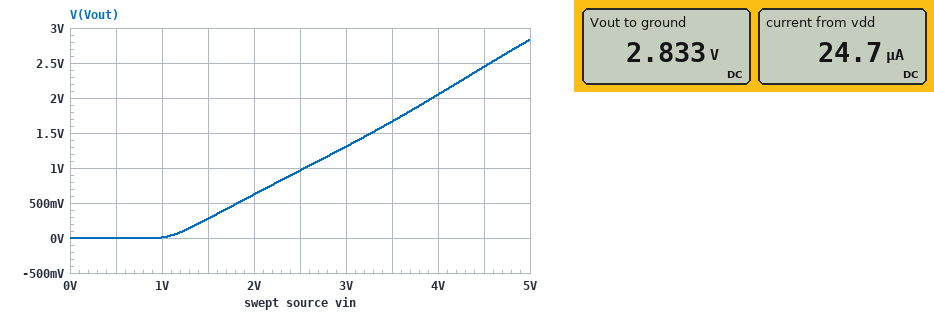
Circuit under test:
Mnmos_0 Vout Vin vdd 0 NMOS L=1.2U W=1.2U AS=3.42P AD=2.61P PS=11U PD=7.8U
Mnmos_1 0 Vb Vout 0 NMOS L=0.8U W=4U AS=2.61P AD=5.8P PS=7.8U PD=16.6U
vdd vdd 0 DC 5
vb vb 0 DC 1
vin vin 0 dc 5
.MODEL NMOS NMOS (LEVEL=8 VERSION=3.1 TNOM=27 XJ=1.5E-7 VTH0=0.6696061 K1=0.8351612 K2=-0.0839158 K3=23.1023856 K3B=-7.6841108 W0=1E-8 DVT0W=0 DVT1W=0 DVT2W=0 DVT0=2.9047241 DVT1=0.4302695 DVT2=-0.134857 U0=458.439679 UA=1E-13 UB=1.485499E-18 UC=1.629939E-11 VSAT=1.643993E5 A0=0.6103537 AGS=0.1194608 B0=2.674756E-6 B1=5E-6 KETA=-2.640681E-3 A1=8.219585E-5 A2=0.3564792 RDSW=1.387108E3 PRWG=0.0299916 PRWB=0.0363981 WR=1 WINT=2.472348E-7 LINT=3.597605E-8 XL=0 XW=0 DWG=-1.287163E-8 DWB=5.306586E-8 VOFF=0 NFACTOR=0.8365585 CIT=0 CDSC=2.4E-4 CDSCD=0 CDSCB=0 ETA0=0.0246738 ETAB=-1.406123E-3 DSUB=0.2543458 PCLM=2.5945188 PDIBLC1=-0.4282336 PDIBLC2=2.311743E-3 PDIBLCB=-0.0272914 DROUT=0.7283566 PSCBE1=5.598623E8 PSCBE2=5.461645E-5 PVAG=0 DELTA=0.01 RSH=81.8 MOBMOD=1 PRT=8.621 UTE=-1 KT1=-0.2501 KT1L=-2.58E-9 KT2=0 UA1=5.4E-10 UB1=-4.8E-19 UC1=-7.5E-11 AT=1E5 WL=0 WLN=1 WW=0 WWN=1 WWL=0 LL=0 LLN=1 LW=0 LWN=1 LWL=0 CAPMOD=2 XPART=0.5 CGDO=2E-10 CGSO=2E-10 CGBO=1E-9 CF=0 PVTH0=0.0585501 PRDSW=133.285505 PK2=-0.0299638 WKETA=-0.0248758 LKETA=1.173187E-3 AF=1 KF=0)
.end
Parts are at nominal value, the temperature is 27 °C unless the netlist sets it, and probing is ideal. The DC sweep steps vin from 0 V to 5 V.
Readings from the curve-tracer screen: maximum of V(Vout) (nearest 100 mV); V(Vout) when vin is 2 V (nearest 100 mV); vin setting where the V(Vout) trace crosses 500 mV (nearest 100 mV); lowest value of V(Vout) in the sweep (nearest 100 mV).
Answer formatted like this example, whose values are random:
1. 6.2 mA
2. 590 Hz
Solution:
1. 2.8 V
2. 600 mV
3. 1.8 V
4. 0 V
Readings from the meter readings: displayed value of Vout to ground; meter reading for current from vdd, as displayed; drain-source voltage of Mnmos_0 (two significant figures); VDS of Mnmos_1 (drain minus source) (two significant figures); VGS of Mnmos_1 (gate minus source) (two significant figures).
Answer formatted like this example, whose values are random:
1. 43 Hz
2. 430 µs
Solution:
1. 2.833 V
2. 24.7 µA
3. -2.2 V
4. -2.8 V
5. -1.8 V
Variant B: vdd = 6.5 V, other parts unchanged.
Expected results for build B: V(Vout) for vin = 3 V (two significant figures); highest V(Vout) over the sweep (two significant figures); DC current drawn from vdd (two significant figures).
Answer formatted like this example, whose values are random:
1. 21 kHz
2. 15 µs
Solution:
1. 1.5 V
2. 2.9 V
3. 25 µA
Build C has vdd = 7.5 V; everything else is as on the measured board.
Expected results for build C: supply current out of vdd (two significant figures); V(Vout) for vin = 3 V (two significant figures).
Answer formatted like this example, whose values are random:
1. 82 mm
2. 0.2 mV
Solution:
1. 27 µA
2. 1.5 V
